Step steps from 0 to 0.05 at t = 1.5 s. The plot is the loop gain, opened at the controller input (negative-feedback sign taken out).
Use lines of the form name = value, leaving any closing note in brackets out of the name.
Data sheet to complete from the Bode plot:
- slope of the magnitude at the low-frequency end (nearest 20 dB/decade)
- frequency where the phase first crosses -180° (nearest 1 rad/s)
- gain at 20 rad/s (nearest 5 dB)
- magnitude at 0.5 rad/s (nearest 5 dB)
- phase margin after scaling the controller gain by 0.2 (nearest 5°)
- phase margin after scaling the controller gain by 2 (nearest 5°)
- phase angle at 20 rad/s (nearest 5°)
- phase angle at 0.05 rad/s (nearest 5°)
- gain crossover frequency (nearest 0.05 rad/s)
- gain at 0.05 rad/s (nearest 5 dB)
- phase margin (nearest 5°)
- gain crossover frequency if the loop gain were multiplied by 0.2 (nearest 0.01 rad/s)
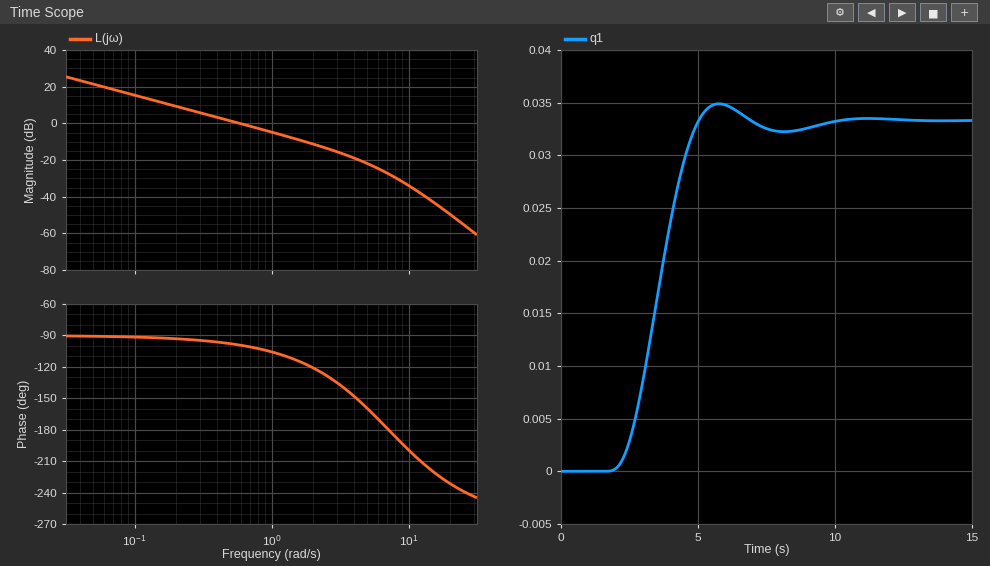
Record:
slope of the magnitude at the low-frequency end = -20 dB/decade
frequency where the phase first crosses -180° = 7 rad/s
gain at 20 rad/s = -50 dB
magnitude at 0.5 rad/s = 0 dB
phase margin after scaling the controller gain by 0.2 = 90°
phase margin after scaling the controller gain by 2 = 70°
phase angle at 20 rad/s = -230°
phase angle at 0.05 rad/s = -90°
gain crossover frequency = 0.60 rad/s
gain at 0.05 rad/s = 20 dB
phase margin = 80°
gain crossover frequency if the loop gain were multiplied by 0.2 = 0.12 rad/s
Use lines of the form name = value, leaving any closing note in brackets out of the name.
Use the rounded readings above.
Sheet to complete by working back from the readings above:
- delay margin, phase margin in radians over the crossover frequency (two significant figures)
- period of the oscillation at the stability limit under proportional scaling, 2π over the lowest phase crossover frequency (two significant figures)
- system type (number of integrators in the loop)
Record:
delay margin, phase margin in radians over the crossover frequency = 2.3 s
period of the oscillation at the stability limit under proportional scaling, 2π over the lowest phase crossover frequency = 0.90 s
system type = 1
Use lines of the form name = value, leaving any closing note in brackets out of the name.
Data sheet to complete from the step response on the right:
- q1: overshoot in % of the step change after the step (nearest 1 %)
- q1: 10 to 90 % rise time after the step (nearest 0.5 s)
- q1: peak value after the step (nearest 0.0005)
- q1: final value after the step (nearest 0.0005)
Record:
q1: overshoot in % of the step change after the step = 5 %
q1: 10 to 90 % rise time after the step = 2.0 s
q1: peak value after the step = 0.0350
q1: final value after the step = 0.0335
